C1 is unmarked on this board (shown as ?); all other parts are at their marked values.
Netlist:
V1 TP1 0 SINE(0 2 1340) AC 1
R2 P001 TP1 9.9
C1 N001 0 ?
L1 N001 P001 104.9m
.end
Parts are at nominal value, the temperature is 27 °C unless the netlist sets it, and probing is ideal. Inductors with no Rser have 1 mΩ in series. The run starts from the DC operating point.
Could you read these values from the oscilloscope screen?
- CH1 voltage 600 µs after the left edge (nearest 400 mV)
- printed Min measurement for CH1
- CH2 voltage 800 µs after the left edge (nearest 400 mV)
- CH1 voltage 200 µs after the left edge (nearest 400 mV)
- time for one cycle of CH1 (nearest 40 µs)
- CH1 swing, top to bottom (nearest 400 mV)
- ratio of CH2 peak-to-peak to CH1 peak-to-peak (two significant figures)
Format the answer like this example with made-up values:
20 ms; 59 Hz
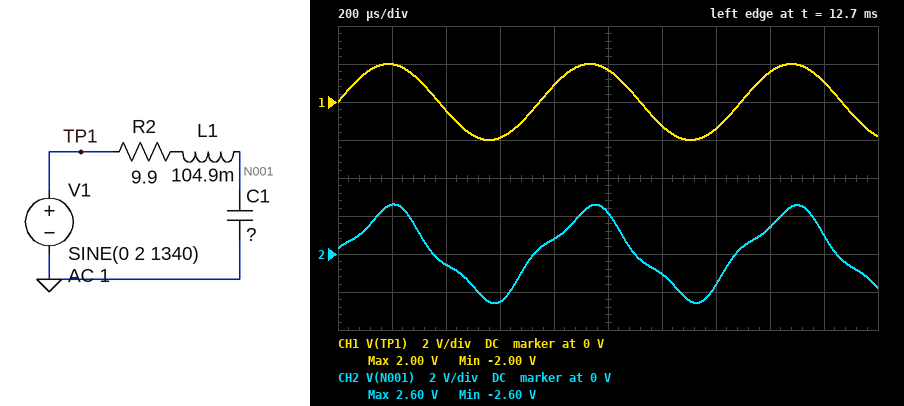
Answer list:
-2.0 V; -2.00 V; 800 mV; 2.0 V; 760 µs; 4.0 V; 1.3
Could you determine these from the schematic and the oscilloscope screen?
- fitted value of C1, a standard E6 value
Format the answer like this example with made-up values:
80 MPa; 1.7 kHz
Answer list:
15 nF
